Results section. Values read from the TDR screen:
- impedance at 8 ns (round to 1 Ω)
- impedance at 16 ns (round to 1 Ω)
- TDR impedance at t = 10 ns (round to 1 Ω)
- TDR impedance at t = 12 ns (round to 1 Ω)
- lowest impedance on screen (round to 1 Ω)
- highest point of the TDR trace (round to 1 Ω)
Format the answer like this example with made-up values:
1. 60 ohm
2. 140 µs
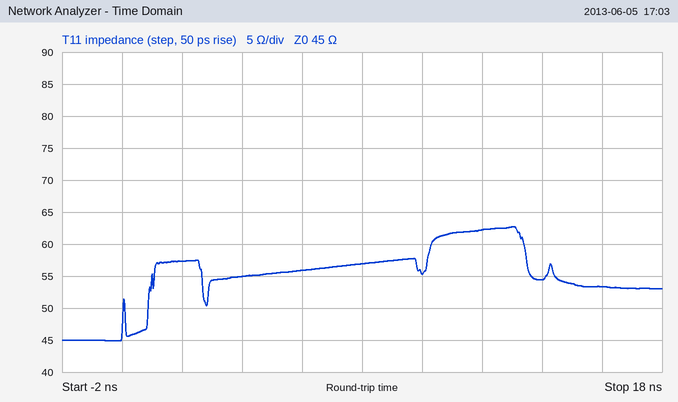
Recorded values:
1. 57 Ω
2. 53 Ω
3. 55 Ω
4. 62 Ω
5. 45 Ω
6. 63 Ω
